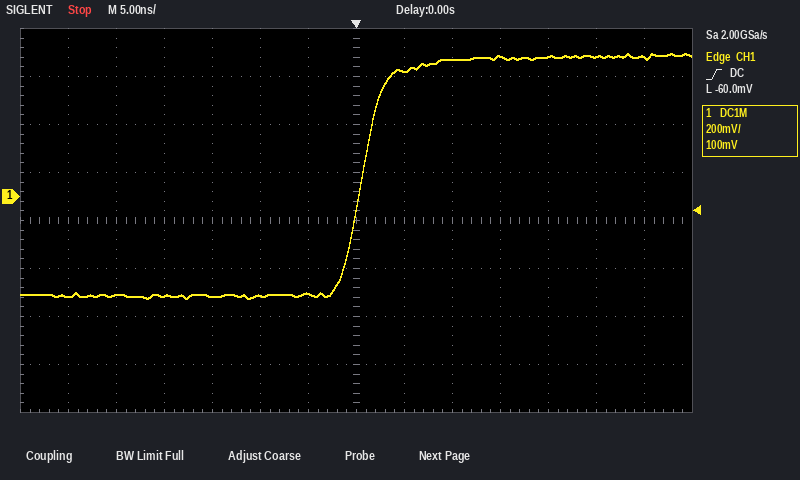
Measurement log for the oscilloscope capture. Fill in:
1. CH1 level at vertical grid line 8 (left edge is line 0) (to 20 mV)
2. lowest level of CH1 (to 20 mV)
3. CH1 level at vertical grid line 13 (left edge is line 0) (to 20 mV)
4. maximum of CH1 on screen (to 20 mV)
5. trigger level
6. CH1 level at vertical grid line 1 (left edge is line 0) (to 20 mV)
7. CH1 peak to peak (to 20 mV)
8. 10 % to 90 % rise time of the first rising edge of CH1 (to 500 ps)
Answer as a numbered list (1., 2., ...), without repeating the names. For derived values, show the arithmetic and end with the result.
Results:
1. 520 mV
2. -420 mV
3. 580 mV
4. 600 mV
5. -60.0 mV
6. -420 mV
7. 600 mV − (-420 mV) = 1.02 V
8. 4.5 ns
